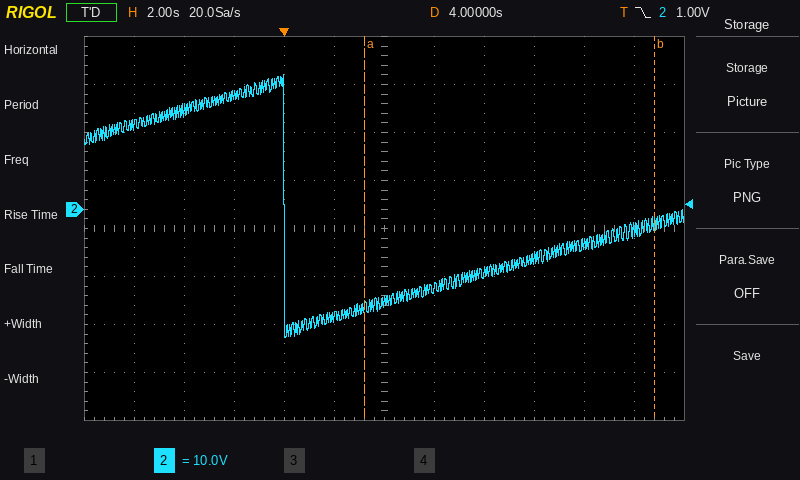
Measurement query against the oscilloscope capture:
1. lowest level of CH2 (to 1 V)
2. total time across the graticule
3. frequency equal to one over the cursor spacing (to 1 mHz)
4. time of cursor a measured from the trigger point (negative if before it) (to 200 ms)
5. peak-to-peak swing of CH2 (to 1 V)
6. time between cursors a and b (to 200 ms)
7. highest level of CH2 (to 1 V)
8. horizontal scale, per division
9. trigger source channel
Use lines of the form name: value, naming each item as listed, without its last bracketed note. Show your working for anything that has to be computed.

lowest level of CH2: -27 V
total time across the graticule: 24 s
frequency equal to one over the cursor spacing: 1 / 11.6 s ≈ 86 mHz
time of cursor a measured from the trigger point (negative if before it): +3.2 s
peak-to-peak swing of CH2: 28 V − (-27 V) = 55 V
time between cursors a and b: 11.6 s
highest level of CH2: 28 V
horizontal scale, per division: 2 s
trigger source channel: CH2
